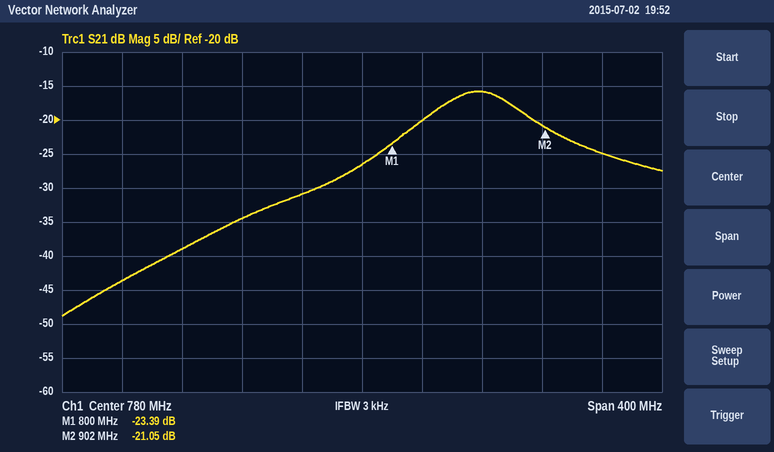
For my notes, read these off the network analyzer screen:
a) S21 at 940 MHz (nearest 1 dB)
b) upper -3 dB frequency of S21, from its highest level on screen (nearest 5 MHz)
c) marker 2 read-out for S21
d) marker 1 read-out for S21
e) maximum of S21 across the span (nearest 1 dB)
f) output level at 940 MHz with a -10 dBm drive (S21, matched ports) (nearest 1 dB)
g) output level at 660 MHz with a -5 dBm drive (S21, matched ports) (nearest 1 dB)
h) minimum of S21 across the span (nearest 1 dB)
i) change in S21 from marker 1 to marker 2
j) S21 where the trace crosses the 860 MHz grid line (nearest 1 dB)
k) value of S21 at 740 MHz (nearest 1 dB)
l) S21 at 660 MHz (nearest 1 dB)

-25 dB
885 MHz
-21.05 dB
-23.39 dB
-16 dB
-35 dBm
-44 dBm
-49 dB
2.34 dB
-16 dB
-31 dB
-39 dB
